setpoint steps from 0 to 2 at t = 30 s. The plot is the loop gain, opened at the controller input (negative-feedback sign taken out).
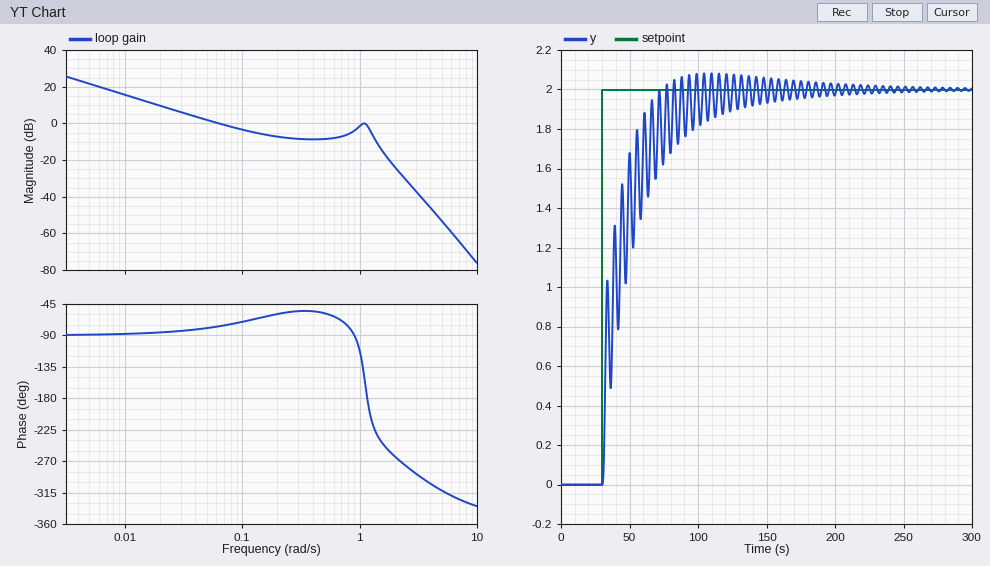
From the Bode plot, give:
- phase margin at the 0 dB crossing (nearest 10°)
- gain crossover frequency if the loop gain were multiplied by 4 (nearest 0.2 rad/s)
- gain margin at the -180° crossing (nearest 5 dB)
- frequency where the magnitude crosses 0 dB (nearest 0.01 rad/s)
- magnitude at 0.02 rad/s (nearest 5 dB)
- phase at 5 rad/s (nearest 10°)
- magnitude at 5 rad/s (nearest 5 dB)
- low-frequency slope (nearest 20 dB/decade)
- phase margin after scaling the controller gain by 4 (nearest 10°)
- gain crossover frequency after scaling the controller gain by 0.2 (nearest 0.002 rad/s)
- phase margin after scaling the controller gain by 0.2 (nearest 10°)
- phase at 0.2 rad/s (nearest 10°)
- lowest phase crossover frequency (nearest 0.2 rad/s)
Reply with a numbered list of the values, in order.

1. 100°
2. 1.4 rad/s
3. 0 dB
4. 0.06 rad/s
5. 10 dB
6. -310°
7. -55 dB
8. -20 dB/decade
9. -60°
10. 0.012 rad/s
11. 90°
12. -60°
13. 1.2 rad/s
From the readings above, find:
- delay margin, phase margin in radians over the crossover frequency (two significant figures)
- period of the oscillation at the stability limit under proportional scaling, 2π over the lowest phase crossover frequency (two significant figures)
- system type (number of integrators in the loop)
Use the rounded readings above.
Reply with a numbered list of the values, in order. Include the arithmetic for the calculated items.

1. 100 × π / 180 / 0.06 = 29 s
2. 2π / 1.2 = 5.2 s
3. 1
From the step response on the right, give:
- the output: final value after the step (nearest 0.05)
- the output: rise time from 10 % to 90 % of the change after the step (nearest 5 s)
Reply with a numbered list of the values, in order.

1. 2.00
2. 30 s
